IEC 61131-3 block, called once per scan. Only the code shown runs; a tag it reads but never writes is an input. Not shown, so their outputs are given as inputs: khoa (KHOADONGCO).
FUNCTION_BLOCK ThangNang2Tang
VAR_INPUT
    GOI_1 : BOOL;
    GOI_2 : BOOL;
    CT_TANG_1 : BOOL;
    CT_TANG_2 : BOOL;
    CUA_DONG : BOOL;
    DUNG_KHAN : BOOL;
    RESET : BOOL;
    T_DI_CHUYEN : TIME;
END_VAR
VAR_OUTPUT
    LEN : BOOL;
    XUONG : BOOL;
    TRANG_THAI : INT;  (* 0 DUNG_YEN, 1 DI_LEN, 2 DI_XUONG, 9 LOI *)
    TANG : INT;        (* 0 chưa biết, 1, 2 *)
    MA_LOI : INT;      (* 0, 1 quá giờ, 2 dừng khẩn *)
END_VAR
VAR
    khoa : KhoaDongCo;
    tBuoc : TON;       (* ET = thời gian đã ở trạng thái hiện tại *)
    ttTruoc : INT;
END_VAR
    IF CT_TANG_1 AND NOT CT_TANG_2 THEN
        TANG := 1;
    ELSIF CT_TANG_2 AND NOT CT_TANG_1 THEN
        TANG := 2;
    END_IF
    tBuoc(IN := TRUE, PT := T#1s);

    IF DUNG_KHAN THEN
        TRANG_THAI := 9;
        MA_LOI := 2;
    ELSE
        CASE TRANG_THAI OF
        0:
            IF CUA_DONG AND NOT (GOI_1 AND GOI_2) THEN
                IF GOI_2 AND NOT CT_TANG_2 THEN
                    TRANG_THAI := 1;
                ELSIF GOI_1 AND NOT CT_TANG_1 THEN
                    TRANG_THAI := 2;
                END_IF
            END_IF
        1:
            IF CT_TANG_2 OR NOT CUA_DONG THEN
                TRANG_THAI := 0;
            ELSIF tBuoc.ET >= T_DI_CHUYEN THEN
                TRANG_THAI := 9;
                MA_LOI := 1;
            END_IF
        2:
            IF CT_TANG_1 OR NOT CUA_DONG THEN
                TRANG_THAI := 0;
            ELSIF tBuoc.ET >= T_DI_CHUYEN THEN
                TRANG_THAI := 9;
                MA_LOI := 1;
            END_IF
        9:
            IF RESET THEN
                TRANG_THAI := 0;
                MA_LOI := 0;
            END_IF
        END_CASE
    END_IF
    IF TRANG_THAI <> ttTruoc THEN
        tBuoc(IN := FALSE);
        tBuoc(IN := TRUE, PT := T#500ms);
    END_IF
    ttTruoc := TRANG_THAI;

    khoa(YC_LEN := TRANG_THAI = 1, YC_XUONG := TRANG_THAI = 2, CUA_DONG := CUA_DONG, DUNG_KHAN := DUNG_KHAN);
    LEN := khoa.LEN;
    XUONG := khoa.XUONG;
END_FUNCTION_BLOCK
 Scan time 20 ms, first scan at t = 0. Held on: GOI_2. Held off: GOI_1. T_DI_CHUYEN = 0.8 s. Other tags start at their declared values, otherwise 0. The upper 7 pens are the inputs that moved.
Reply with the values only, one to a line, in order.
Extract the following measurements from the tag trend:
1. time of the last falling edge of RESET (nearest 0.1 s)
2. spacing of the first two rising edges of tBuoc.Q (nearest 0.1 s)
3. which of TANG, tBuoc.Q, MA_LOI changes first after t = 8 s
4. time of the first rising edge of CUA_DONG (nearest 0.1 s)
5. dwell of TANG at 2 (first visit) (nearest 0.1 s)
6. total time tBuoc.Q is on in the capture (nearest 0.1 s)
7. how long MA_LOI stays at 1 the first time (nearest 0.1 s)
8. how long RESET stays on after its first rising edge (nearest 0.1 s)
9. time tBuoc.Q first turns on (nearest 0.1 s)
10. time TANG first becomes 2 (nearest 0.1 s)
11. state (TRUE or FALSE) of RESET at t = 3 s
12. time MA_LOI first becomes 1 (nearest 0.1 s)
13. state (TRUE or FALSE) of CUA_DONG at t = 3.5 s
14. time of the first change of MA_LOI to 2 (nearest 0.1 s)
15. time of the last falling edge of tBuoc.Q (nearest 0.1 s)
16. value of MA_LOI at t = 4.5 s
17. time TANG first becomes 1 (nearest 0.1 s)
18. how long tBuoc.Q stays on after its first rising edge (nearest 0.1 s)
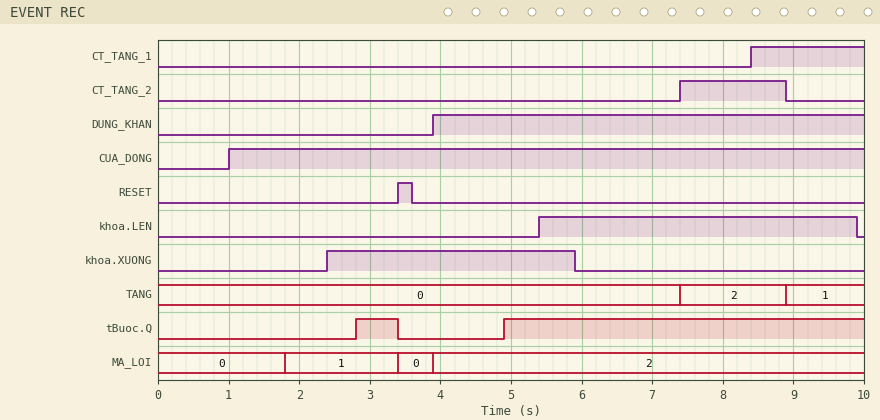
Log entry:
3.6 s
2.1 s
TANG
1.0 s
1.5 s
5.7 s
1.6 s
0.2 s
2.8 s
7.4 s
FALSE
1.8 s
TRUE
3.9 s
3.4 s
2
8.9 s
0.6 s
